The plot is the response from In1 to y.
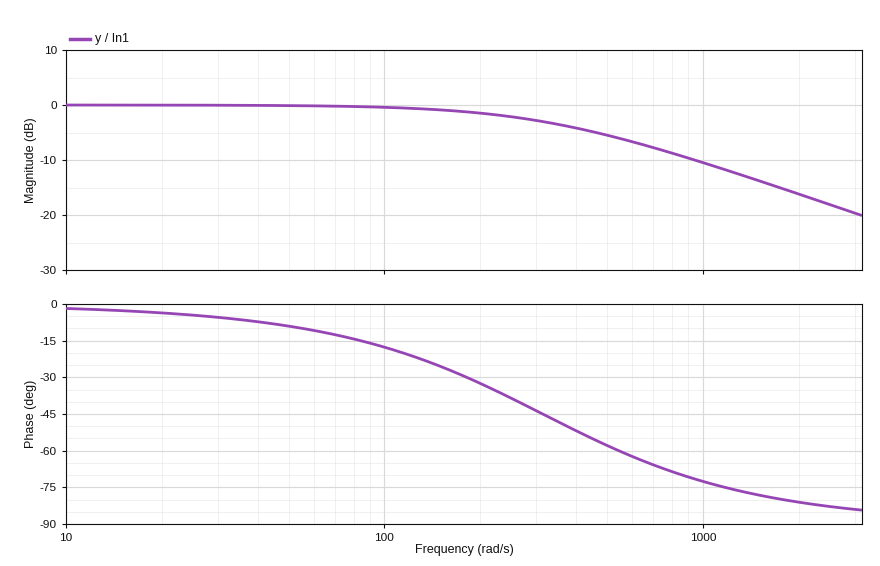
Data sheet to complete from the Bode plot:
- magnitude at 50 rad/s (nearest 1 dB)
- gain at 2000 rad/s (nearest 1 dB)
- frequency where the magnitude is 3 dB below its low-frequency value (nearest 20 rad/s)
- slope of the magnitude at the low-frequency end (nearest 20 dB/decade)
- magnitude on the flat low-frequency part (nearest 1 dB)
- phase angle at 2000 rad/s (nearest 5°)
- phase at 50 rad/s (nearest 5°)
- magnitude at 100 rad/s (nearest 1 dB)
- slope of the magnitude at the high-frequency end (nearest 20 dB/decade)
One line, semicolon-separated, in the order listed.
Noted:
0 dB; -16 dB; 320 rad/s; 0 dB/decade; 0 dB; -80°; -10°; 0 dB; -20 dB/decade
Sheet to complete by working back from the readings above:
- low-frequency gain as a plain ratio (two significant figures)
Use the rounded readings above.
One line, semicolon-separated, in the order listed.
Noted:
1.0
